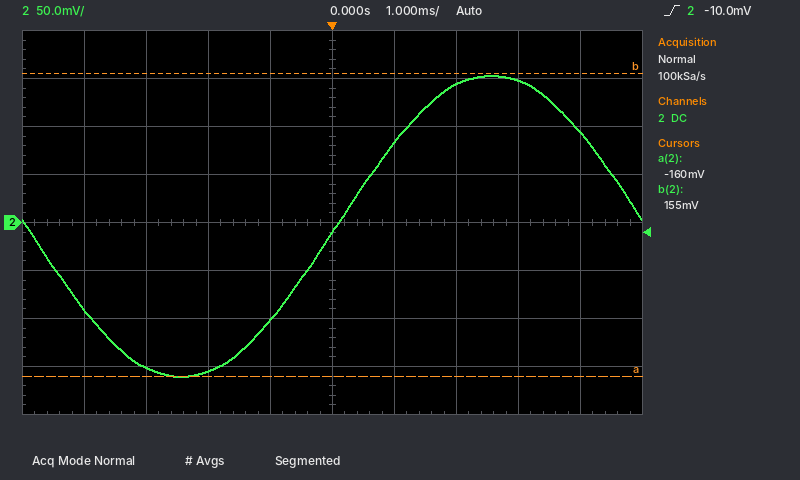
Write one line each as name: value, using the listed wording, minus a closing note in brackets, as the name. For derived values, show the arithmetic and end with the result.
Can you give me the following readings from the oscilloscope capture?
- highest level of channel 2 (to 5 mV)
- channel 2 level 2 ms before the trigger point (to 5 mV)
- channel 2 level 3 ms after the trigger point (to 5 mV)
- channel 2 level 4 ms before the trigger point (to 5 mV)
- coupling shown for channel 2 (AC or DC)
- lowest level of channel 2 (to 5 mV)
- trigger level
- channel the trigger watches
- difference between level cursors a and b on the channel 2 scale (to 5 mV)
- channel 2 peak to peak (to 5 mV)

highest level of channel 2: 155 mV
channel 2 level 2 ms before the trigger point: -155 mV
channel 2 level 3 ms after the trigger point: 150 mV
channel 2 level 4 ms before the trigger point: -90 mV
coupling shown for channel 2: DC
lowest level of channel 2: -160 mV
trigger level: -10.0 mV
channel the trigger watches: channel 2
difference between level cursors a and b on the channel 2 scale: 315 mV
channel 2 peak to peak: 155 mV − (-160 mV) = 315 mV
